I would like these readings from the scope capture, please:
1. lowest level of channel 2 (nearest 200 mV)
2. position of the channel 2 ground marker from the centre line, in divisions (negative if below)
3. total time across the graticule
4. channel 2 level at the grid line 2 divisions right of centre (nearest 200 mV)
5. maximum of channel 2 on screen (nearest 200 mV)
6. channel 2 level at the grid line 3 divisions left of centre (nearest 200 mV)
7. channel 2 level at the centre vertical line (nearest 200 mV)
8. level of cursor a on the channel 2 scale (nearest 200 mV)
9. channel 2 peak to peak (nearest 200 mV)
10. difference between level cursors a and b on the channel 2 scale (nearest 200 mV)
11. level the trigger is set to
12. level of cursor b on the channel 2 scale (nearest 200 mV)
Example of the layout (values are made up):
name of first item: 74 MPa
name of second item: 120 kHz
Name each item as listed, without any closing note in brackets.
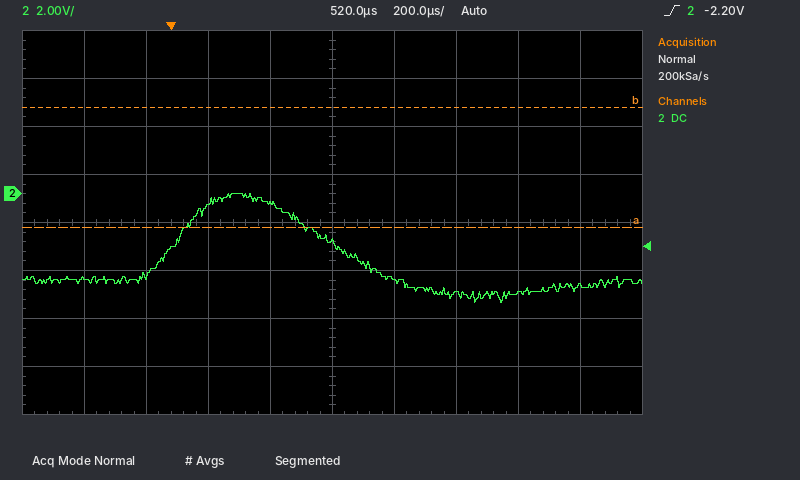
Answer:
lowest level of channel 2: -4.6 V
position of the channel 2 ground marker from the centre line, in divisions: +0.6 div
total time across the graticule: 2 ms
channel 2 level at the grid line 2 divisions right of centre: -4.2 V
maximum of channel 2 on screen: 0.0 V
channel 2 level at the grid line 3 divisions left of centre: -3.4 V
channel 2 level at the centre vertical line: -2.0 V
level of cursor a on the channel 2 scale: -1.4 V
channel 2 peak to peak: 4.6 V
difference between level cursors a and b on the channel 2 scale: 5.0 V
level the trigger is set to: -2.20 V
level of cursor b on the channel 2 scale: 3.6 V
